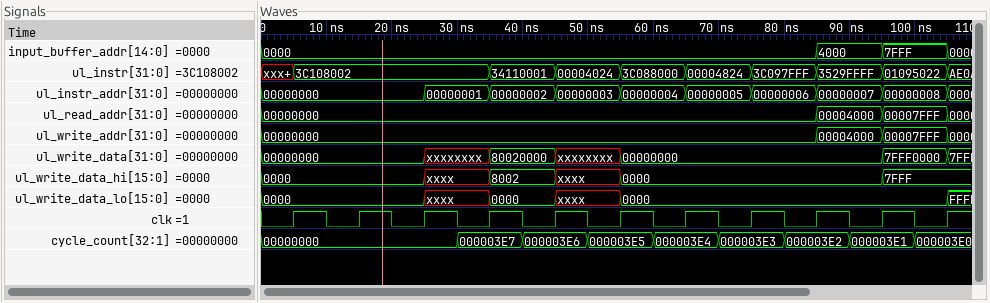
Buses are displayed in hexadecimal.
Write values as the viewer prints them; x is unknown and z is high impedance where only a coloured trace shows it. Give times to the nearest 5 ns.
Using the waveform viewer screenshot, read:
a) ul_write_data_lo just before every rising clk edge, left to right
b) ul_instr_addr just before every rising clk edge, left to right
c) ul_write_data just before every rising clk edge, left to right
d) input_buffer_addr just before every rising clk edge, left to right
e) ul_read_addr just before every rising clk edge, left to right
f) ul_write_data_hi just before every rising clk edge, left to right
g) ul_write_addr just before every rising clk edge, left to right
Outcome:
0000, 0000, 0000, xxxx, 0000, xxxx, 0000, 0000, 0000, 0000, 0000
00000000, 00000000, 00000000, 00000001, 00000002, 00000003, 00000004, 00000005, 00000006, 00000007, 00000008
00000000, 00000000, 00000000, xxxxxxxx, 80020000, xxxxxxxx, 00000000, 00000000, 00000000, 00000000, 7FFF0000
0000, 0000, 0000, 0000, 0000, 0000, 0000, 0000, 0000, 4000, 7FFF
00000000, 00000000, 00000000, 00000000, 00000000, 00000000, 00000000, 00000000, 00000000, 00004000, 00007FFF
0000, 0000, 0000, xxxx, 8002, xxxx, 0000, 0000, 0000, 0000, 7FFF
00000000, 00000000, 00000000, 00000000, 00000000, 00000000, 00000000, 00000000, 00000000, 00004000, 00007FFF
